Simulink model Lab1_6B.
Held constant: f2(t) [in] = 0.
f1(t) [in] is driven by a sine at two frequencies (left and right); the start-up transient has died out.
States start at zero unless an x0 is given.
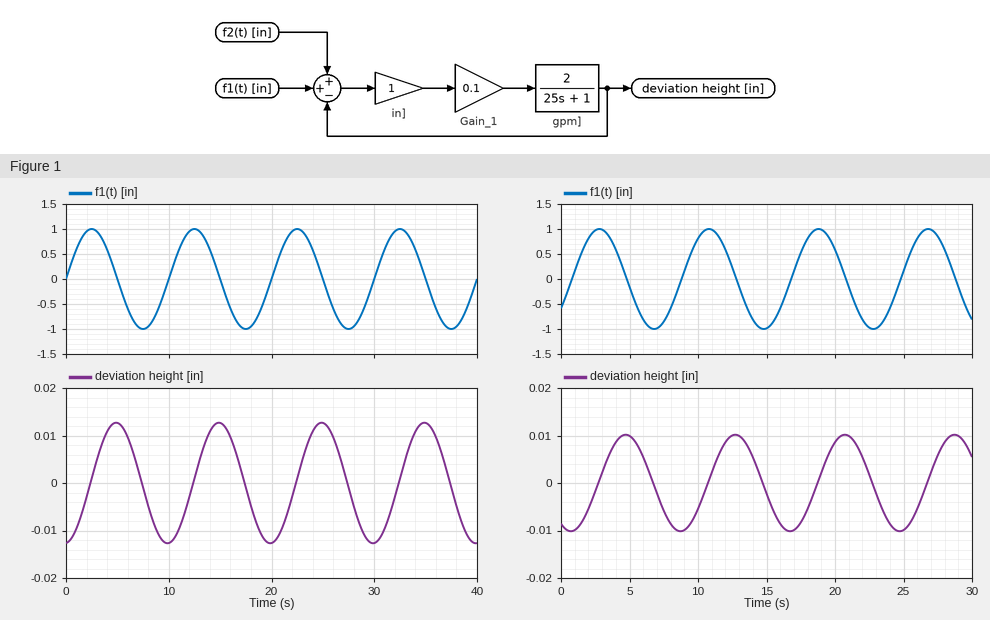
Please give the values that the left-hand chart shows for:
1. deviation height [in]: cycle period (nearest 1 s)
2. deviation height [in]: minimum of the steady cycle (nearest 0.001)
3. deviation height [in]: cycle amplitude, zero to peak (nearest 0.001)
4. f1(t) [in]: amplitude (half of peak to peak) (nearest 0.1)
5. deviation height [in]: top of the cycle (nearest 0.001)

10 s
-0.013
0.013
1.0
0.013
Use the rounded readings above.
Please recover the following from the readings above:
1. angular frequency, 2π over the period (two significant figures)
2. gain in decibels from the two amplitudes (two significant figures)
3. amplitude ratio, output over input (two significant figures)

0.63 rad/s
-38 dB
0.013
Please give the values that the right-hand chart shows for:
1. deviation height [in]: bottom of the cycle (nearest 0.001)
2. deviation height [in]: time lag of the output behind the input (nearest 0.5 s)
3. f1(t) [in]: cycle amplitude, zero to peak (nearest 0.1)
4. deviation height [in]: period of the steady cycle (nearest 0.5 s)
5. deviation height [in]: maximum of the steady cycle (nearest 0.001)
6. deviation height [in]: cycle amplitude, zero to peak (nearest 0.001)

-0.010
2.0 s
1.0
8.0 s
0.010
0.010
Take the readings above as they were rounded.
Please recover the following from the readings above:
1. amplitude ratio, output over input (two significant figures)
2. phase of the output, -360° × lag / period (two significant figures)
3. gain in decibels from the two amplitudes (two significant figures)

0.010
-90°
-40 dB
